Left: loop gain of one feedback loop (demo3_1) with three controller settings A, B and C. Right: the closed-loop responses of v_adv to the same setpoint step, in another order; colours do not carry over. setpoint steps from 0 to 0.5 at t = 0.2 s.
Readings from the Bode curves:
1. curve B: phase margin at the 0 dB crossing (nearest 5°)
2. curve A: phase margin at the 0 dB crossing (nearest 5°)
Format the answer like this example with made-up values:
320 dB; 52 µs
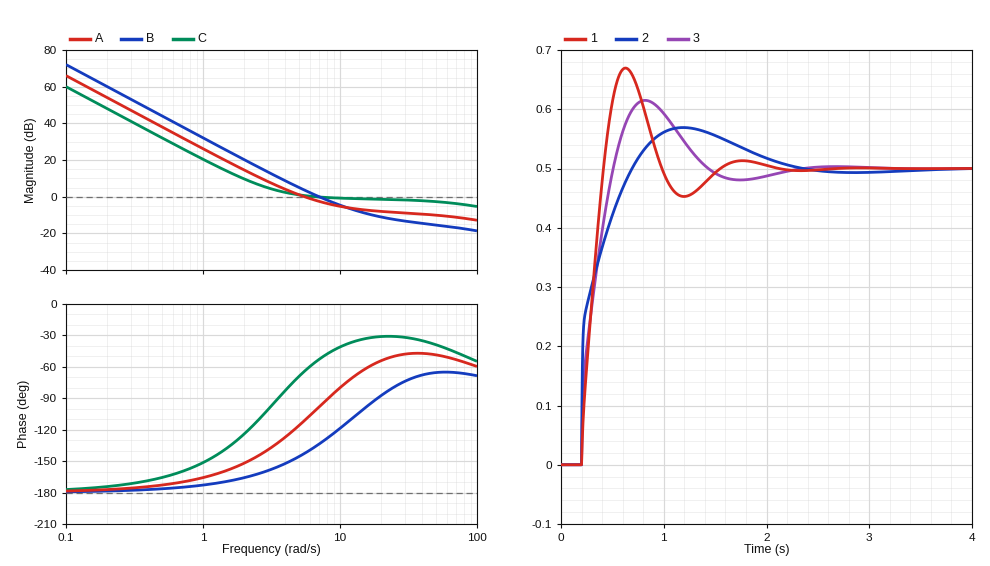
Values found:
45°; 70°
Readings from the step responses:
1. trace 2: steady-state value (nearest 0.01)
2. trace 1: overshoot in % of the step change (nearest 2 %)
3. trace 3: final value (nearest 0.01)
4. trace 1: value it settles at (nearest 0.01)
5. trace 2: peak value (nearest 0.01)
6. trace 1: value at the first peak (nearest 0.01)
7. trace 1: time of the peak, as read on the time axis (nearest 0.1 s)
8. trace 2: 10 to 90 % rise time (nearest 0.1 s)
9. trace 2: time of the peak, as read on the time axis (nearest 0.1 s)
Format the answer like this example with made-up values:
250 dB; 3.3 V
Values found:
0.50; 34 %; 0.50; 0.50; 0.57; 0.67; 0.6 s; 0.4 s; 1.2 s
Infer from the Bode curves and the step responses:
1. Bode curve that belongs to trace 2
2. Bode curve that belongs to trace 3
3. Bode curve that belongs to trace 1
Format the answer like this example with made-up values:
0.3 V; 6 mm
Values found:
C; A; B
